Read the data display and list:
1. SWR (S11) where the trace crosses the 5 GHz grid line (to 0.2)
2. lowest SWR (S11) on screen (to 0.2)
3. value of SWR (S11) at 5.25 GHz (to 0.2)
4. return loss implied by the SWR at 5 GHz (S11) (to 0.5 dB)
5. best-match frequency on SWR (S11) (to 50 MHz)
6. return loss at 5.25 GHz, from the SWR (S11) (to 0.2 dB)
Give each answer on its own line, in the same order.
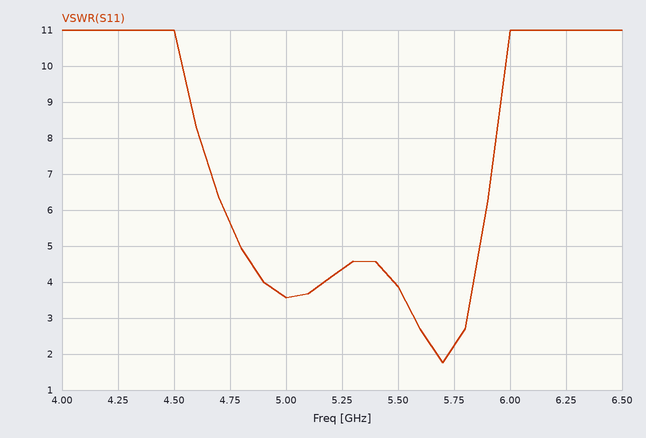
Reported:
3.6
1.8
4.4
5.0 dB
5.70 GHz
4.0 dB
